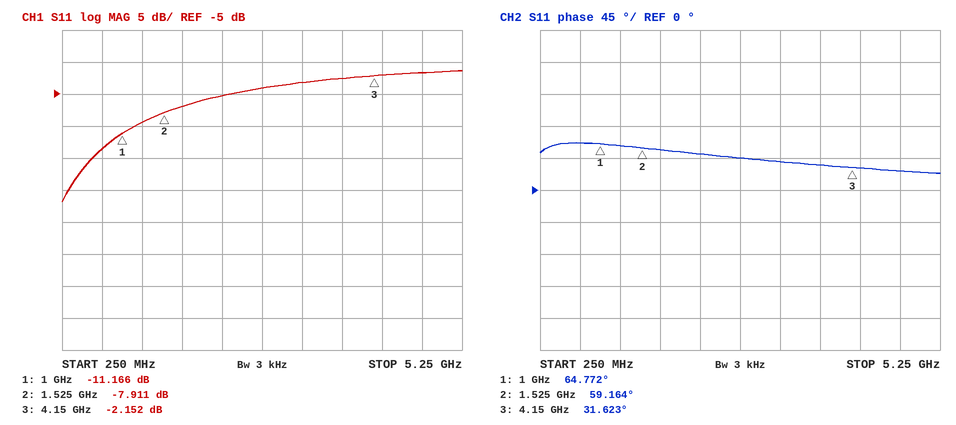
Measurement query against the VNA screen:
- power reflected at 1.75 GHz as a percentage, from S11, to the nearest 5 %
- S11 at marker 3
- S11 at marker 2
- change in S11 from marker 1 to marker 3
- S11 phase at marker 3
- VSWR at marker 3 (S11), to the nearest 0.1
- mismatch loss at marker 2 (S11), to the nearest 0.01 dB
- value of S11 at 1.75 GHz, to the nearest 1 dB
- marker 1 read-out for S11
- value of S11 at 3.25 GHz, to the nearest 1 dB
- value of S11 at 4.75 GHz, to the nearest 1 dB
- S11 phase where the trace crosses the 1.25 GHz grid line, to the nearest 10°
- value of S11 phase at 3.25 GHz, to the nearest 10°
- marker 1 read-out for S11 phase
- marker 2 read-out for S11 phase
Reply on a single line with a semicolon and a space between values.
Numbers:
20 %; -2.152 dB; -7.911 dB; 9.014 dB; 31.623°; 8.1; 0.77 dB; -7 dB; -11.166 dB; -3 dB; -2 dB; 60°; 40°; 64.772°; 59.164°
